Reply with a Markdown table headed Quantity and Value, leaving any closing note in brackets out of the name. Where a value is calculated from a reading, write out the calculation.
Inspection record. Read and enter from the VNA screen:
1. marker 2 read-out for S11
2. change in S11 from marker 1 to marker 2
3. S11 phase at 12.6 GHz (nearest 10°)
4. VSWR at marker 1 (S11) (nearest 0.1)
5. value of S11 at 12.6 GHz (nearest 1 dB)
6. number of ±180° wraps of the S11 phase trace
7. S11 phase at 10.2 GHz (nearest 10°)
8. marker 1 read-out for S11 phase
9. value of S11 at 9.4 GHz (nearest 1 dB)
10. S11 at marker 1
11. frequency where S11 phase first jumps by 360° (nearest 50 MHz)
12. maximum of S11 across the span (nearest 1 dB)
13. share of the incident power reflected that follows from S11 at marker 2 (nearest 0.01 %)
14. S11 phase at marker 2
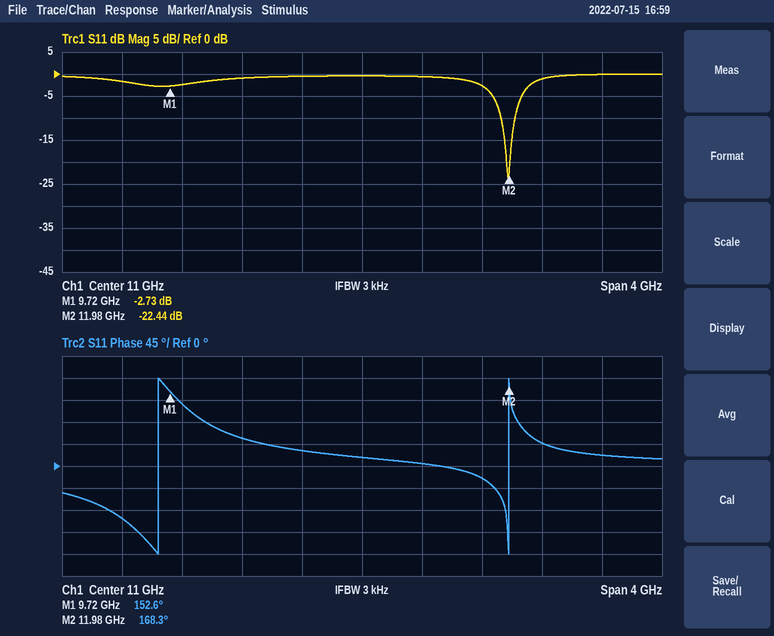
| Quantity | Value |
|---|---|
| marker 2 read-out for S11 | -22.44 dB |
| change in S11 from marker 1 to marker 2 | -22.44 − (-2.73) = -19.71 dB |
| S11 phase at 12.6 GHz | 20° |
| VSWR at marker 1 (S11) | (1 + 0.7303)/(1 − 0.7303) ≈ 6.4 |
| value of S11 at 12.6 GHz | 0 dB |
| number of ±180° wraps of the S11 phase trace | 2 |
| S11 phase at 10.2 GHz | 60° |
| marker 1 read-out for S11 phase | 152.6° |
| value of S11 at 9.4 GHz | -2 dB |
| S11 at marker 1 | -2.73 dB |
| frequency where S11 phase first jumps by 360° | 9.65 GHz |
| maximum of S11 across the span | 0 dB |
| share of the incident power reflected that follows from S11 at marker 2 | 10^(-22.44/10) ≈ 0.57 % |
| S11 phase at marker 2 | 168.3° |
